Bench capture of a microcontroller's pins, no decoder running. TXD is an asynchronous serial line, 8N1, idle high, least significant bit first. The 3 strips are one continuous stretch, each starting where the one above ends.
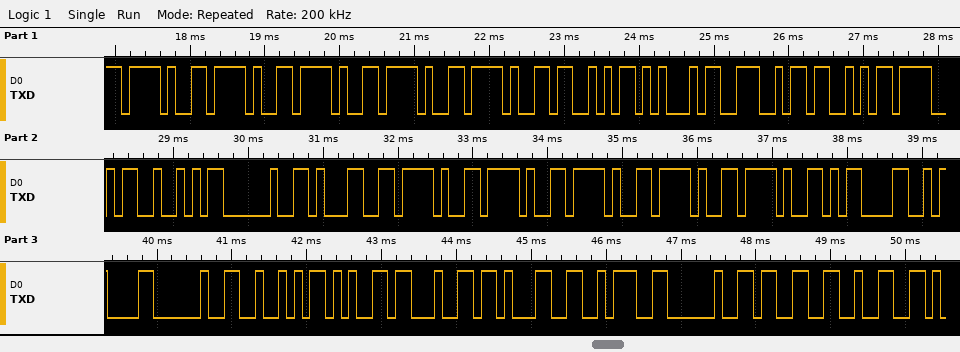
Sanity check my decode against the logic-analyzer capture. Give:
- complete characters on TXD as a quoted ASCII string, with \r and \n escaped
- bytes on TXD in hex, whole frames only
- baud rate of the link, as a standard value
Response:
"/////SENSOR 1/////\r\n Red1: 32"
0x2F 0x2F 0x2F 0x2F 0x2F 0x53 0x45 0x4E 0x53 0x4F 0x52 0x20 0x31 0x2F 0x2F 0x2F 0x2F 0x2F 0x0D 0x0A 0x20 0x52 0x65 0x64 0x31 0x3A 0x20 0x33 0x32
9600 baud
